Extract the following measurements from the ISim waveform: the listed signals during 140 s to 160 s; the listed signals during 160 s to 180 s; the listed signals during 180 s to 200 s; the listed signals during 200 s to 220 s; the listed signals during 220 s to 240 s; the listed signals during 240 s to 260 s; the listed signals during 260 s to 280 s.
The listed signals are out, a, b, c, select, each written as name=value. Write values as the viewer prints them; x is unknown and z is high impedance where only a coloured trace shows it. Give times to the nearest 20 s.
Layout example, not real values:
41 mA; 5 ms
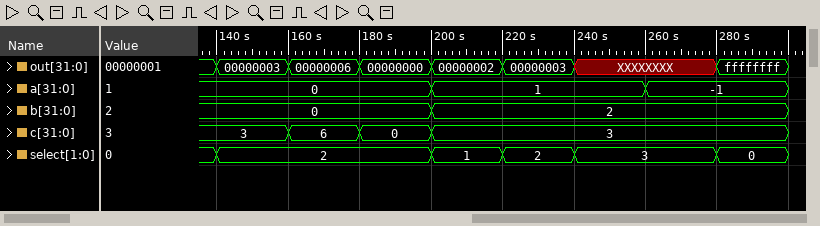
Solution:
out=00000003, a=0, b=0, c=3, select=2; out=00000006, a=0, b=0, c=6, select=2; out=00000000, a=0, b=0, c=0, select=2; out=00000002, a=1, b=2, c=3, select=1; out=00000003, a=1, b=2, c=3, select=2; out=XXXXXXXX, a=1, b=2, c=3, select=3; out=XXXXXXXX, a=-1, b=2, c=3, select=3
